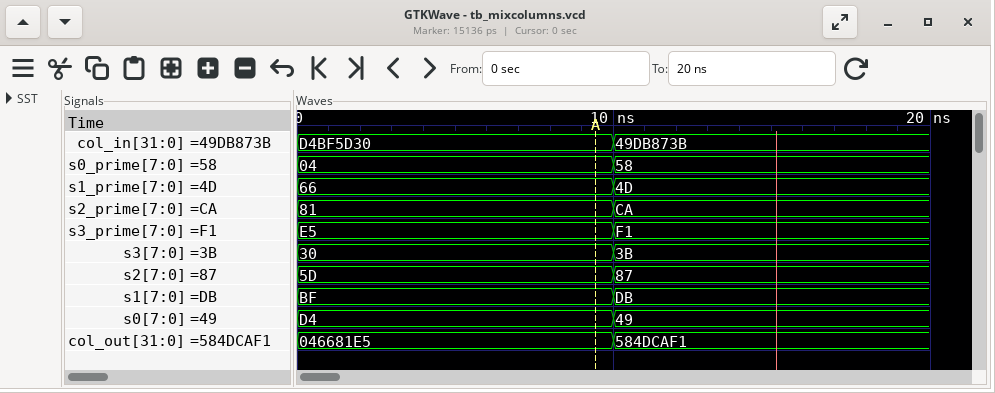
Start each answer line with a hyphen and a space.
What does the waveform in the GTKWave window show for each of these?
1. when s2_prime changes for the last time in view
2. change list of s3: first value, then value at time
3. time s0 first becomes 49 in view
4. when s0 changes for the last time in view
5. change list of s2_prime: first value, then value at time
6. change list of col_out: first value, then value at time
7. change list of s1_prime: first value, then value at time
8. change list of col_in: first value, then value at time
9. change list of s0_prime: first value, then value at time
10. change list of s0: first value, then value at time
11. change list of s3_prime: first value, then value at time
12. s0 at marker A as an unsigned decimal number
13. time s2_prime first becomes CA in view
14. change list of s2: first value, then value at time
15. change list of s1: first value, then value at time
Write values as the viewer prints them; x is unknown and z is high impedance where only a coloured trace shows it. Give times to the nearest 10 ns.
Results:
- 10 ns
- 30, 3B at 10 ns
- 10 ns
- 10 ns
- 81, CA at 10 ns
- 046681E5, 584DCAF1 at 10 ns
- 66, 4D at 10 ns
- D4BF5D30, 49DB873B at 10 ns
- 04, 58 at 10 ns
- D4, 49 at 10 ns
- E5, F1 at 10 ns
- 212
- 10 ns
- 5D, 87 at 10 ns
- BF, DB at 10 ns
